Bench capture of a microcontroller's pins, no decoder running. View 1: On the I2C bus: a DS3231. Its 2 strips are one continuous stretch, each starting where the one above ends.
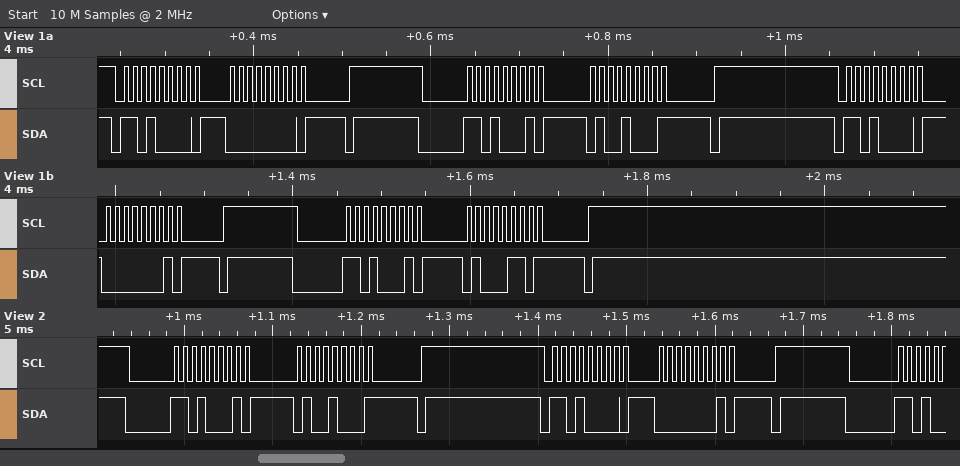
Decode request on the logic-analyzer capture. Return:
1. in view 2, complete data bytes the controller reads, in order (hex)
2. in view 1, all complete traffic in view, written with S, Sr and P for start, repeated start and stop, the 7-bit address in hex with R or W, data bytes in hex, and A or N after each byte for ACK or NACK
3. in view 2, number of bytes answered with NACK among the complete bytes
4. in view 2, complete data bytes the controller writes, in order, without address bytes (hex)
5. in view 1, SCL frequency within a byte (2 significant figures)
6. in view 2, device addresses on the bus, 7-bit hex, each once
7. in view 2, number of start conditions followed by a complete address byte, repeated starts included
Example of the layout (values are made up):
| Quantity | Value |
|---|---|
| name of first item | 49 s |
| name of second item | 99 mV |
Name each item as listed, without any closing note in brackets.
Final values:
| Quantity | Value |
|---|---|
| in view 2, complete data bytes the controller reads, in order | 48 |
| in view 1, all complete traffic in view, written with S, Sr and P for start, repeated start and stop, the 7-bit address in hex with R or W, data bytes in hex, and A or N after each byte for ACK or NACK | S 68W A 00 A P S 68R A 48 N P S 68W A 01 A P S 68R A 46 N P |
| in view 2, number of bytes answered with NACK among the complete bytes | 1 |
| in view 2, complete data bytes the controller writes, in order, without address bytes | 01 |
| in view 1, SCL frequency within a byte | 100 kHz |
| in view 2, device addresses on the bus, 7-bit hex, each once | 0x68 |
| in view 2, number of start conditions followed by a complete address byte, repeated starts included | 2 |
